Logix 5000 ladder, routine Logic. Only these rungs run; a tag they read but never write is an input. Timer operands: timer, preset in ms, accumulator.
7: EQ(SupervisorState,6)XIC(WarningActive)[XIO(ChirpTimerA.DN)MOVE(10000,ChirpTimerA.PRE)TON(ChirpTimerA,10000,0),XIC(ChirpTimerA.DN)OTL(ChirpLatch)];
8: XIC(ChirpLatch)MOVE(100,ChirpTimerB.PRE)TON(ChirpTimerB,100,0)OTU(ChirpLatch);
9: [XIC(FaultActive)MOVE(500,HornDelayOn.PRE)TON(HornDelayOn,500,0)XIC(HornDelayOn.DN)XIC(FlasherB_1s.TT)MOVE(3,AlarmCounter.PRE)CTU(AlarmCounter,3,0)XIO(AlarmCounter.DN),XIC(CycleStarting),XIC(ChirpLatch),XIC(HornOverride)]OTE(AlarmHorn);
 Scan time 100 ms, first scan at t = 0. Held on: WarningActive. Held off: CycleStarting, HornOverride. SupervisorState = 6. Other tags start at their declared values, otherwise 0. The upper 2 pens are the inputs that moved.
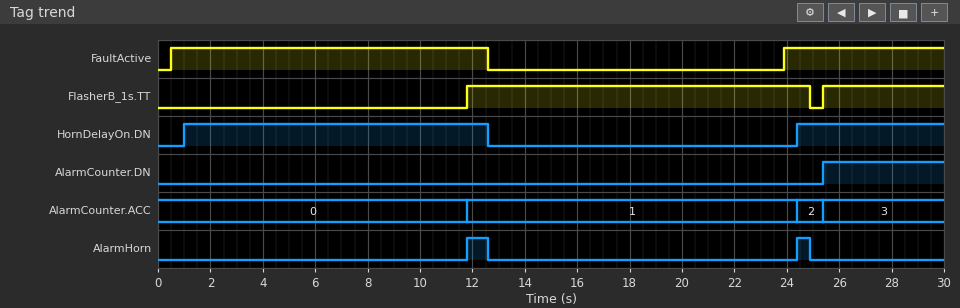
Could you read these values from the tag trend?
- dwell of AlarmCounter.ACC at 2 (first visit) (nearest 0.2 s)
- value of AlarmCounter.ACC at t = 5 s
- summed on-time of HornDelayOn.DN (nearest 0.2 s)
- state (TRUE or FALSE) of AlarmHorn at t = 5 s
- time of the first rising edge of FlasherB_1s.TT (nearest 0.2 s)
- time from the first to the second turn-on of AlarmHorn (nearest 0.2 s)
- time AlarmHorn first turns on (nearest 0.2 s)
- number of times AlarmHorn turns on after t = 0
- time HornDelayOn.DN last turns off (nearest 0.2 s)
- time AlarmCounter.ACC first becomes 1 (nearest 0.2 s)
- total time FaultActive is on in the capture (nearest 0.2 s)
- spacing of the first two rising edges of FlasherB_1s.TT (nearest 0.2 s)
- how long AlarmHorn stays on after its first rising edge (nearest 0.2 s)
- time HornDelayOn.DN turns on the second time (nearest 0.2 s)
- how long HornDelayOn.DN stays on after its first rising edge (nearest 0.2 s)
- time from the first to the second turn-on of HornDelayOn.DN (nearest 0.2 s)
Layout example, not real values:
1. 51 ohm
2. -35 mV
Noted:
1. 1.0 s
2. 0
3. 17.2 s
4. FALSE
5. 11.8 s
6. 12.6 s
7. 11.8 s
8. 2
9. 12.6 s
10. 11.8 s
11. 18.2 s
12. 13.6 s
13. 0.8 s
14. 24.4 s
15. 11.6 s
16. 23.4 s
